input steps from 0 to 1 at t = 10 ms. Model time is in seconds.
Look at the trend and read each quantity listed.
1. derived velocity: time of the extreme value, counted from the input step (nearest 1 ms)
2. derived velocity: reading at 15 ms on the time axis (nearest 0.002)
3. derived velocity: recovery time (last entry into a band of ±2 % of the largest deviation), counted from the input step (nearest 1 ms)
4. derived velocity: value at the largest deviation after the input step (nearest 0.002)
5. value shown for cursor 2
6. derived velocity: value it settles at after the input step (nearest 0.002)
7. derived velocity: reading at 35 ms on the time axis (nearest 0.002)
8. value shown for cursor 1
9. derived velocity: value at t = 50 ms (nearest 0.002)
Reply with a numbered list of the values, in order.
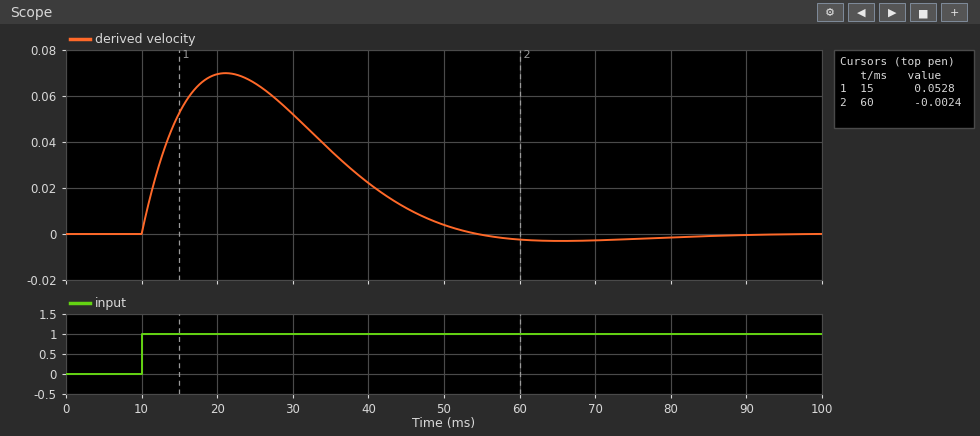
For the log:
1. 11 ms
2. 0.052
3. 71 ms
4. 0.070
5. -0.0024
6. 0.000
7. 0.036
8. 0.0528
9. 0.004
